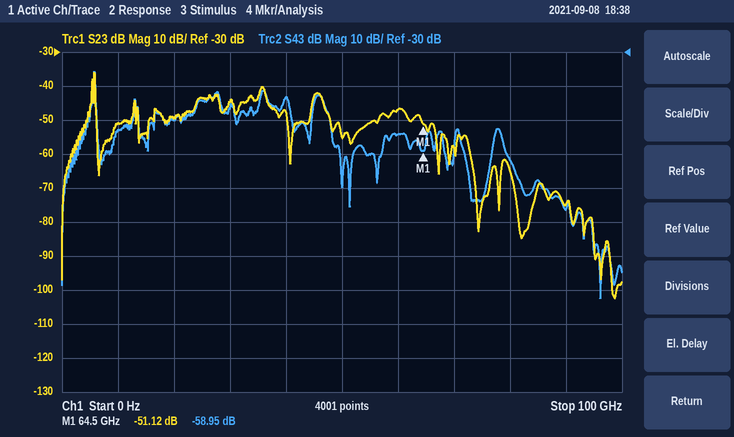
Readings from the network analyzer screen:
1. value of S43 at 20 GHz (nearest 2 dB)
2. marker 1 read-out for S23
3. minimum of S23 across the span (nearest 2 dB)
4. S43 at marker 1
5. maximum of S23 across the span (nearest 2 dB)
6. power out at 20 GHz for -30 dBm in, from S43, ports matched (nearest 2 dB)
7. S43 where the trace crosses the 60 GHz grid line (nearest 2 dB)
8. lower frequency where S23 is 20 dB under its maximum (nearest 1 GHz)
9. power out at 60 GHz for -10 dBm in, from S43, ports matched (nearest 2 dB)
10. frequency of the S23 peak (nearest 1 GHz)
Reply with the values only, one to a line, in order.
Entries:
-50 dB
-51.12 dB
-102 dB
-58.95 dB
-36 dB
-80 dBm
-54 dB
3 GHz
-64 dBm
6 GHz
